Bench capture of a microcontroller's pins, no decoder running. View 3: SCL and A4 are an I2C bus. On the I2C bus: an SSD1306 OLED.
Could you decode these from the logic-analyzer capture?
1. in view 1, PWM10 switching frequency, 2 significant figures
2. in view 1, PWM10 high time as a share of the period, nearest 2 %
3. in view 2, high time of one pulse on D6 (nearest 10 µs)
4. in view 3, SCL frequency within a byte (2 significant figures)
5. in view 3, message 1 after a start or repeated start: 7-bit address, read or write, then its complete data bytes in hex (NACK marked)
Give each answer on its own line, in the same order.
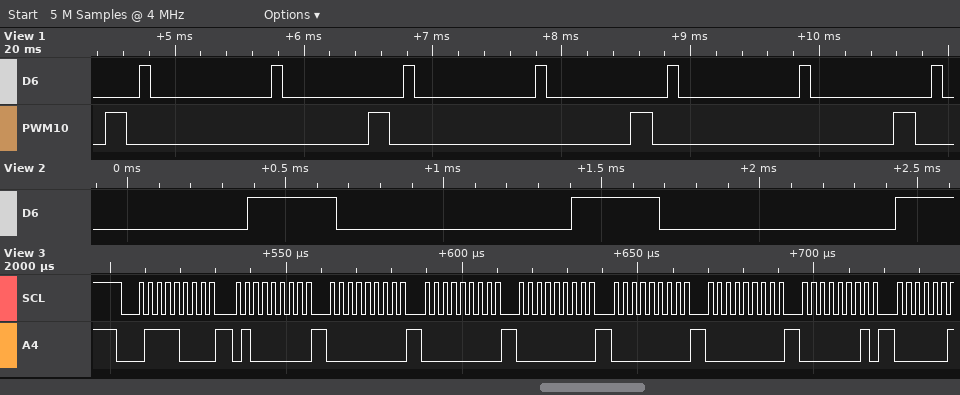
490 Hz
8 %
280 µs
400 kHz
0x3C write: 40 00 00 00 00 00 01
